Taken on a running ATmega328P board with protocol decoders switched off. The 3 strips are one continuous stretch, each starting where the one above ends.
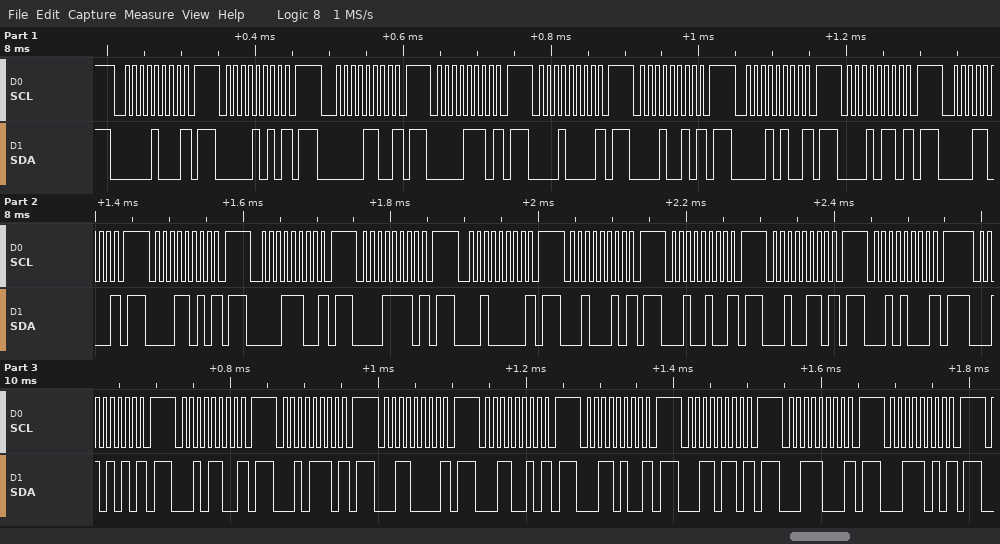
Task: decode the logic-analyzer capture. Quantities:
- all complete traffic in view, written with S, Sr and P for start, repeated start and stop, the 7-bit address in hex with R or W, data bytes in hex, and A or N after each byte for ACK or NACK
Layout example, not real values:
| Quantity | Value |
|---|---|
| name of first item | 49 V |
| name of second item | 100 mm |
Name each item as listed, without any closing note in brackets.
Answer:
| Quantity | Value |
|---|---|
| all complete traffic in view, written with S, Sr and P for start, repeated start and stop, the 7-bit address in hex with R or W, data bytes in hex, and A or N after each byte for ACK or NACK | S 04W N P S 05W N P S 06W N P S 07W N P S 08W N P S 09W N P S 0AW N P S 0BW N P S 0CW N P S 0DW N P S 0EW N P S 0FW N P S 10W N P S 11W N P S 12W N P S 13W N P S 14W N P S 15W N P S 16W N P S 17W N P S 18W N P S 19W N P S 1AW N P S 1BW N P S 1CW N P S 1DW N P |
